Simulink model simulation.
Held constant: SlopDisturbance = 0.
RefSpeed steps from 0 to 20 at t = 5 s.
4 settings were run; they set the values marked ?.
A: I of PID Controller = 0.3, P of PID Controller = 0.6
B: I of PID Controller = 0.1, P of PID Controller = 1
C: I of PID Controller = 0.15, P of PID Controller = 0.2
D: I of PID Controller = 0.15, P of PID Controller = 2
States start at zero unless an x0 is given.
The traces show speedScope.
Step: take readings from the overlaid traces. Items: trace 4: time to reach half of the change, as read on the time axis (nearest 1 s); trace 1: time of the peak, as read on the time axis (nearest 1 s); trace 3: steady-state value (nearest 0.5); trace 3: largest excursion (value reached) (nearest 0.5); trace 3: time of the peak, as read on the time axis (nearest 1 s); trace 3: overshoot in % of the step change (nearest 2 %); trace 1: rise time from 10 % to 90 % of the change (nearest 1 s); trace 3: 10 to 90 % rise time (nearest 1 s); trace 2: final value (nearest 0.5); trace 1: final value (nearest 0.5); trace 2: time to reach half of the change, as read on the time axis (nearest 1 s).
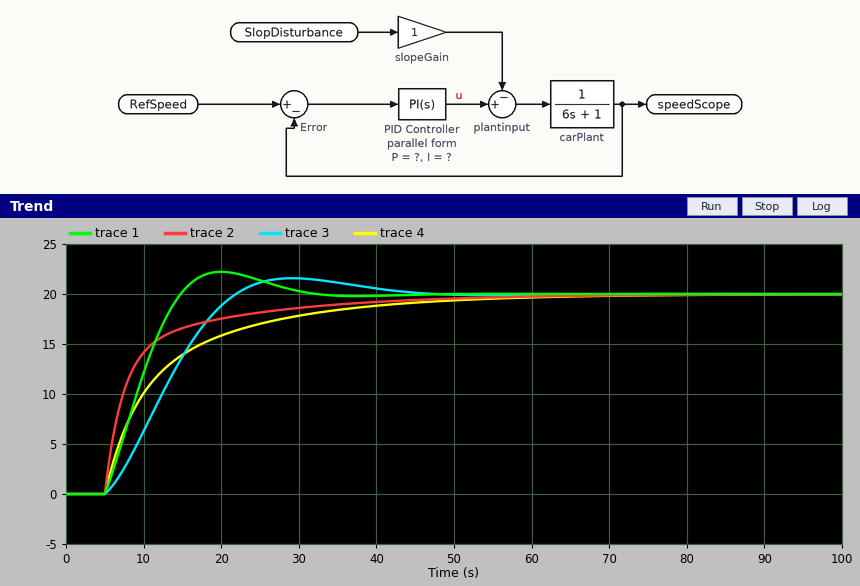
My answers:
10 s
20 s
20.0
21.5
29 s
8 %
7 s
12 s
20.0
20.0
7 s
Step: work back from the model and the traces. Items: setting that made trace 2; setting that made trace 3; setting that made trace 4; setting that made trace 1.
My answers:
D
C
B
A
